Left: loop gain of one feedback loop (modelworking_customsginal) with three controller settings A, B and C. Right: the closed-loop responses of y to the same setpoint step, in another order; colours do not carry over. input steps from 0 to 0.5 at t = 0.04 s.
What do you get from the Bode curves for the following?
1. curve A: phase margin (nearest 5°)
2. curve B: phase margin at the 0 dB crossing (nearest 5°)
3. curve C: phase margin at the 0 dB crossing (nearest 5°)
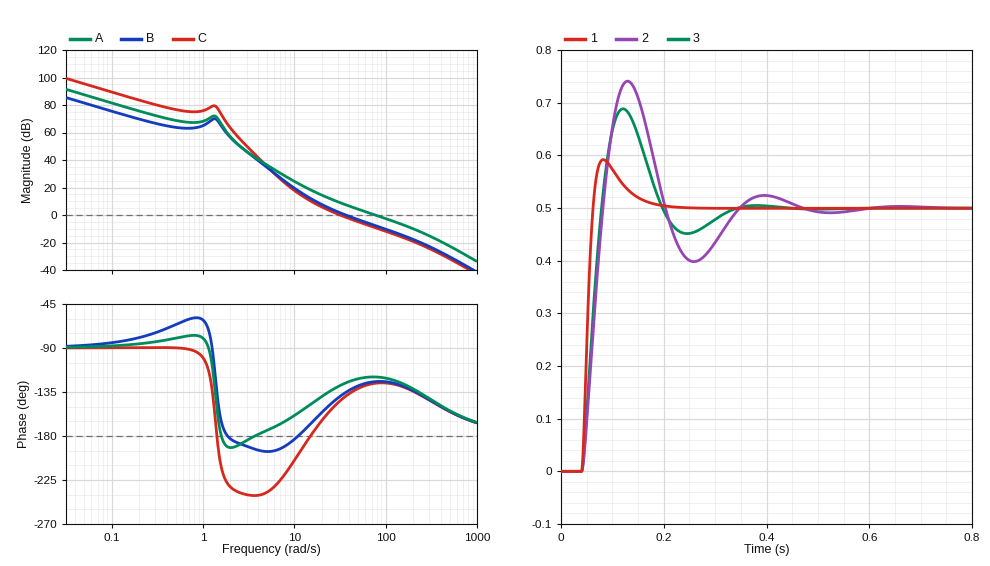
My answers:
60°
45°
35°
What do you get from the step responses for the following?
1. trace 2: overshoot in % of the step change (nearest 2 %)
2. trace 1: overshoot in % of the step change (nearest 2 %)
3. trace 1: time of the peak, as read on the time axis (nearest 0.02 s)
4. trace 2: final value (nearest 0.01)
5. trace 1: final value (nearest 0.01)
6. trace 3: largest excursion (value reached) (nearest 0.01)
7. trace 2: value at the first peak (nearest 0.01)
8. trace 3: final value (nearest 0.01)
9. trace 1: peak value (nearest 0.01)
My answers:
48 %
18 %
0.08 s
0.50
0.50
0.69
0.74
0.50
0.59
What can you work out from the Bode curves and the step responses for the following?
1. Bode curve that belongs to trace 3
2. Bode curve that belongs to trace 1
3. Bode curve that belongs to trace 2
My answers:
B
A
C
